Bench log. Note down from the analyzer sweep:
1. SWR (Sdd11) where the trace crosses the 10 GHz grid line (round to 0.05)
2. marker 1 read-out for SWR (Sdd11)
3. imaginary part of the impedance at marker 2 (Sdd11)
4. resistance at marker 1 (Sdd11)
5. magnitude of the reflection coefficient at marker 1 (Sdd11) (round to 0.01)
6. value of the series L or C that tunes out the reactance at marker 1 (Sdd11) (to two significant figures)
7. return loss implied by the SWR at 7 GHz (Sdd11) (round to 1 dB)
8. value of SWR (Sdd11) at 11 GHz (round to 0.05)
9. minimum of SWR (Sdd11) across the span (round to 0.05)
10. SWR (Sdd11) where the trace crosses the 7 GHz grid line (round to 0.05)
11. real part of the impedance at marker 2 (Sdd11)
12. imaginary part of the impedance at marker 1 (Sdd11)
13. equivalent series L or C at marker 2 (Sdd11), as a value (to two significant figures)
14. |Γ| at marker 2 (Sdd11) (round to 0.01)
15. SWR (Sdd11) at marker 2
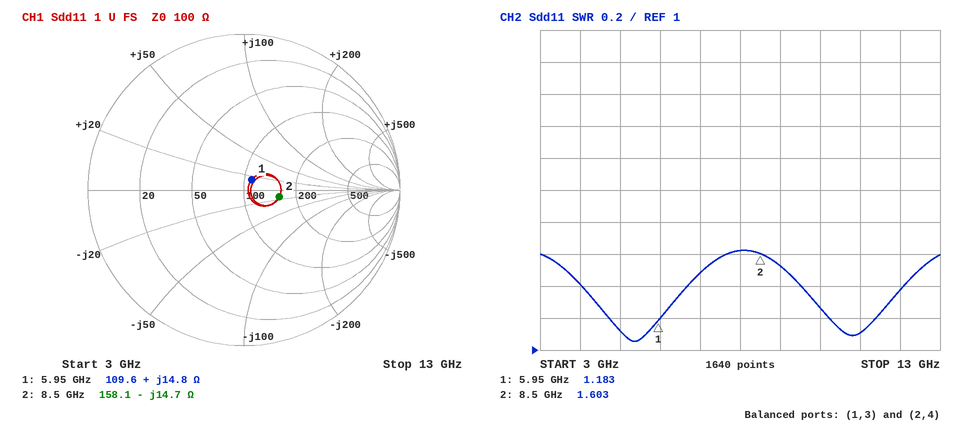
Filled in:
1.25
1.183
-14.7 Ω
109.6 Ω
0.08
1.8 pF
14 dB
1.10
1.05
1.50
158.1 Ω
+14.8 Ω
1.3 pF
0.23
1.603
